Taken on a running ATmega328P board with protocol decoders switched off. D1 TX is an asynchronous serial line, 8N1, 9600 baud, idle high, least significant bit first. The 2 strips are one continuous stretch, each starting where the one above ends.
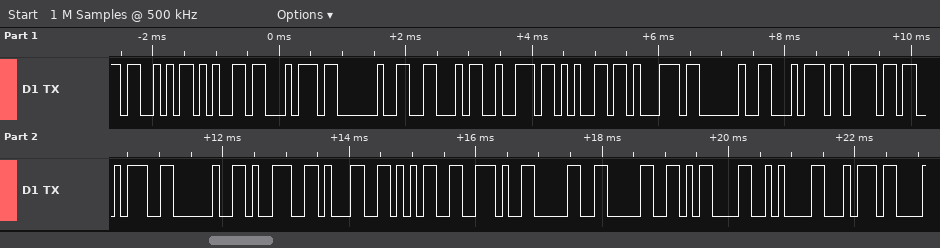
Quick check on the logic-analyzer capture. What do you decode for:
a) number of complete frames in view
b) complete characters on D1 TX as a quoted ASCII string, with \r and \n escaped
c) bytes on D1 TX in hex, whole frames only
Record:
22
"Set Freq to: 915.00\r\nt"
53 65 74 20 46 72 65 71 20 74 6F 3A 20 39 31 35 2E 30 30 0D 0A 74
